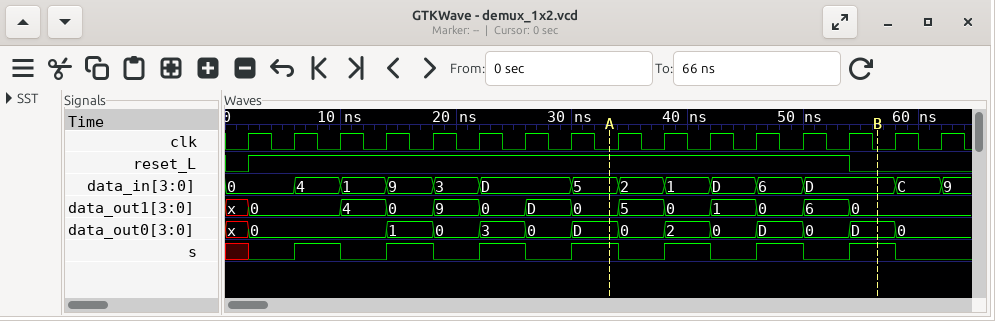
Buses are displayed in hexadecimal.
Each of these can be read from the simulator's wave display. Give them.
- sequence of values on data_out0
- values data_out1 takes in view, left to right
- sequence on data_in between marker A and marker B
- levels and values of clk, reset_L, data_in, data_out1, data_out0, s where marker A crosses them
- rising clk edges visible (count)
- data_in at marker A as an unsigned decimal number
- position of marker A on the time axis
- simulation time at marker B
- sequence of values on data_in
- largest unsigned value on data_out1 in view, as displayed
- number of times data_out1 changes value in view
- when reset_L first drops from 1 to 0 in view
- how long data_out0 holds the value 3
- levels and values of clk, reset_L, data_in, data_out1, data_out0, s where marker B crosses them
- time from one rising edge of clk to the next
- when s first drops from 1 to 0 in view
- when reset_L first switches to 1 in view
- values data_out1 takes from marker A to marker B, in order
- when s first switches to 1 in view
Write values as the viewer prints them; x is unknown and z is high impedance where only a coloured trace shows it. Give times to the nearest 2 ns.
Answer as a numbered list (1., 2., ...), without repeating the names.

1. x, 0, 1, 0, 3, 0, D, 0, 2, 0, D, 0, D, 0
2. x, 0, 4, 0, 9, 0, D, 0, 5, 0, 1, 0, 6, 0
3. 5, 2, 1, D, 6, D
4. clk=0, reset_L=1, data_in=5, data_out1=0, data_out0=D, s=1
5. 16
6. 5
7. 34 ns
8. 56 ns
9. 0, 4, 1, 9, 3, D, 5, 2, 1, D, 6, D, C, 9
10. D
11. 13
12. 54 ns
13. 4 ns
14. clk=0, reset_L=0, data_in=D, data_out1=0, data_out0=D, s=1
15. 4 ns
16. 10 ns
17. 2 ns
18. 0, 5, 0, 1, 0, 6, 0
19. 6 ns
